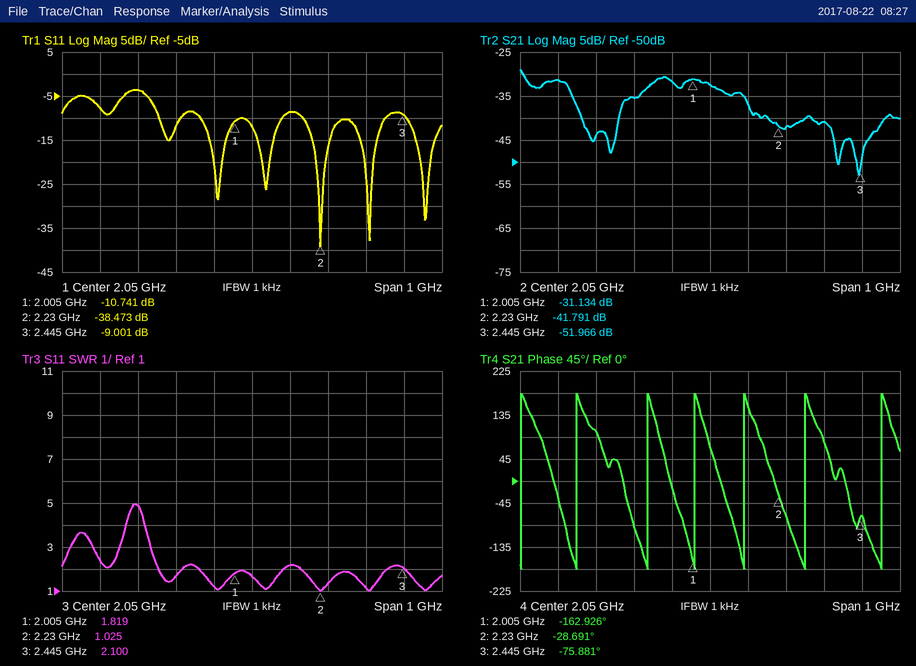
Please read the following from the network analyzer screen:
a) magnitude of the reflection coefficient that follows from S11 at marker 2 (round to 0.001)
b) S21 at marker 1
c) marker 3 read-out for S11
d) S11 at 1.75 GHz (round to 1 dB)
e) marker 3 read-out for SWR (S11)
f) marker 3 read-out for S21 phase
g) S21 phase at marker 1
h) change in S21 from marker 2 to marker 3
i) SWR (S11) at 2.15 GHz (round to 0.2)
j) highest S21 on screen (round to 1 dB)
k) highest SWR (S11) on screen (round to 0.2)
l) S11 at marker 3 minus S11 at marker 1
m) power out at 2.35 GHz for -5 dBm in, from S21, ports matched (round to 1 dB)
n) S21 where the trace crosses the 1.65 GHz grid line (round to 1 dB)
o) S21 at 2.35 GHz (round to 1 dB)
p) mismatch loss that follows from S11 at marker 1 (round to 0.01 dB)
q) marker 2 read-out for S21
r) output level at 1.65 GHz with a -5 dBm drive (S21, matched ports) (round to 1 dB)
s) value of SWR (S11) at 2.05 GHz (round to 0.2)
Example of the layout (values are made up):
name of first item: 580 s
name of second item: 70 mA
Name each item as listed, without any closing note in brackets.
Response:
magnitude of the reflection coefficient that follows from S11 at marker 2: 0.012
S21 at marker 1: -31.134 dB
marker 3 read-out for S11: -9.001 dB
S11 at 1.75 GHz: -4 dB
marker 3 read-out for SWR: 2.100
marker 3 read-out for S21 phase: -75.881°
S21 phase at marker 1: -162.926°
change in S21 from marker 2 to marker 3: -10.175 dB
SWR (S11) at 2.15 GHz: 2.2
highest S21 on screen: -29 dB
highest SWR (S11) on screen: 5.0
S11 at marker 3 minus S11 at marker 1: 1.740 dB
power out at 2.35 GHz for -5 dBm in, from S21, ports matched: -46 dBm
S21 where the trace crosses the 1.65 GHz grid line: -31 dB
S21 at 2.35 GHz: -41 dB
mismatch loss that follows from S11 at marker 1: 0.38 dB
marker 2 read-out for S21: -41.791 dB
output level at 1.65 GHz with a -5 dBm drive (S21, matched ports): -36 dBm
value of SWR (S11) at 2.05 GHz: 1.6
